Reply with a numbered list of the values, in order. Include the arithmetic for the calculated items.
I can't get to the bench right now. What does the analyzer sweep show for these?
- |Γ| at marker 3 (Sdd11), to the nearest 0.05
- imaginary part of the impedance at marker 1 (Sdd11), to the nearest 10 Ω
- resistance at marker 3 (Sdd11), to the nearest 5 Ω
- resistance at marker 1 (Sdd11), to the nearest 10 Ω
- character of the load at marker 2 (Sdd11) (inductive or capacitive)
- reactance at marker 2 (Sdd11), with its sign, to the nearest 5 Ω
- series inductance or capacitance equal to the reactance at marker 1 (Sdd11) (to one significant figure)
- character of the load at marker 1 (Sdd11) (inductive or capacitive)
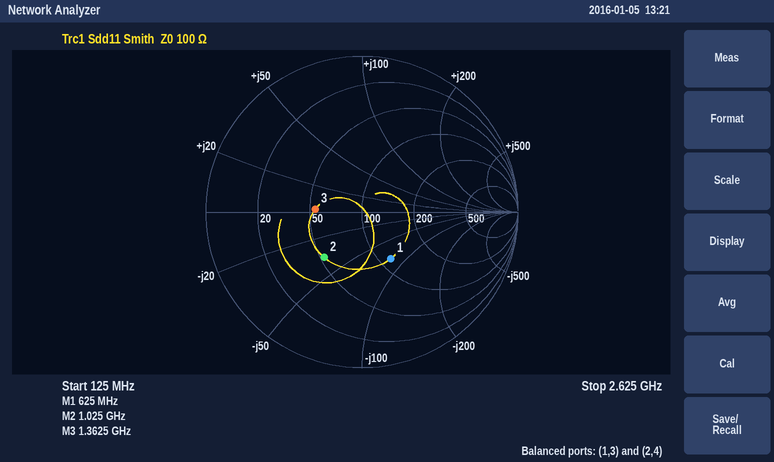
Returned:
1. 0.30
2. -80 Ω
3. 55 Ω
4. 120 Ω
5. capacitive
6. -35 Ω
7. C = 1/(2π × 625 MHz × 80 Ω) ≈ 3 pF
8. capacitive
